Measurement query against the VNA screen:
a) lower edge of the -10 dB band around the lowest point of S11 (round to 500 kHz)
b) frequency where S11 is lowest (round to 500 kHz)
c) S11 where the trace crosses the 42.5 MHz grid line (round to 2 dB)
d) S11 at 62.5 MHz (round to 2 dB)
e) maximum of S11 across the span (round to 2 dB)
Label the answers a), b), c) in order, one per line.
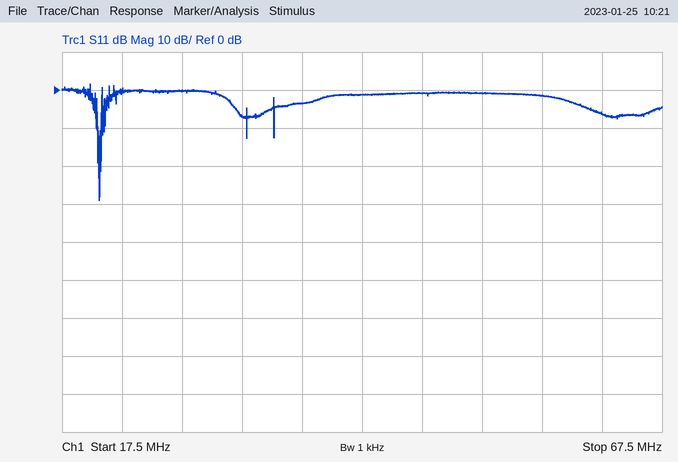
a) 20.5 MHz
b) 20.5 MHz
c) -2 dB
d) -6 dB
e) 2 dB
